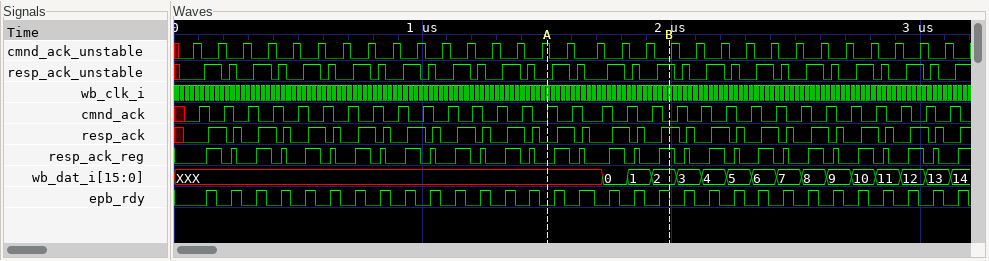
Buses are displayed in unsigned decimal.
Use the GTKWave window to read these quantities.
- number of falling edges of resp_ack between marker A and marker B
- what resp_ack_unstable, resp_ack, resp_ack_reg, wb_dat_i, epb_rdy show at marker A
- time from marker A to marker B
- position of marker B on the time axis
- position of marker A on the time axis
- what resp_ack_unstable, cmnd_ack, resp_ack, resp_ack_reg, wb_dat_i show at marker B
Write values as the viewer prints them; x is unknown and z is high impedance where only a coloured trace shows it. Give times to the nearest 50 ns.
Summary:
4
resp_ack_unstable=0, resp_ack=0, resp_ack_reg=0, wb_dat_i=XXX, epb_rdy=0
500 ns
2000 ns
1500 ns
resp_ack_unstable=1, cmnd_ack=0, resp_ack=1, resp_ack_reg=1, wb_dat_i=2
